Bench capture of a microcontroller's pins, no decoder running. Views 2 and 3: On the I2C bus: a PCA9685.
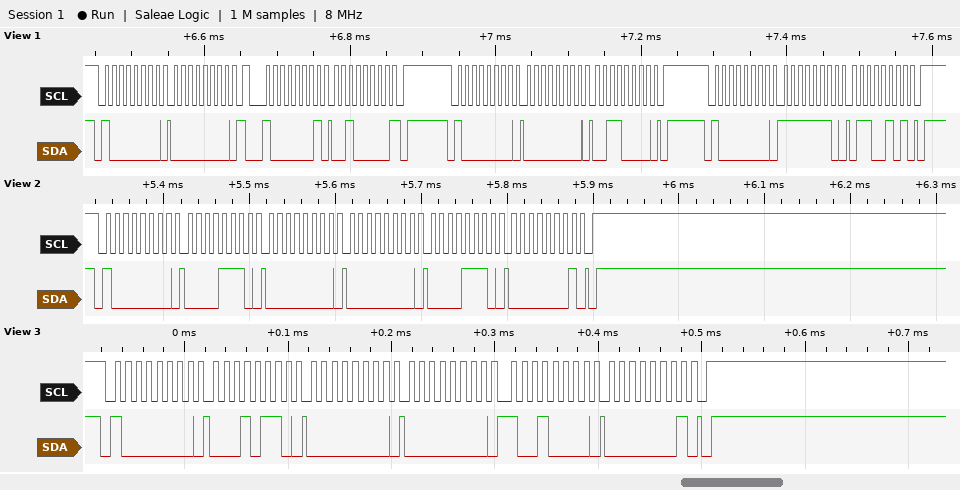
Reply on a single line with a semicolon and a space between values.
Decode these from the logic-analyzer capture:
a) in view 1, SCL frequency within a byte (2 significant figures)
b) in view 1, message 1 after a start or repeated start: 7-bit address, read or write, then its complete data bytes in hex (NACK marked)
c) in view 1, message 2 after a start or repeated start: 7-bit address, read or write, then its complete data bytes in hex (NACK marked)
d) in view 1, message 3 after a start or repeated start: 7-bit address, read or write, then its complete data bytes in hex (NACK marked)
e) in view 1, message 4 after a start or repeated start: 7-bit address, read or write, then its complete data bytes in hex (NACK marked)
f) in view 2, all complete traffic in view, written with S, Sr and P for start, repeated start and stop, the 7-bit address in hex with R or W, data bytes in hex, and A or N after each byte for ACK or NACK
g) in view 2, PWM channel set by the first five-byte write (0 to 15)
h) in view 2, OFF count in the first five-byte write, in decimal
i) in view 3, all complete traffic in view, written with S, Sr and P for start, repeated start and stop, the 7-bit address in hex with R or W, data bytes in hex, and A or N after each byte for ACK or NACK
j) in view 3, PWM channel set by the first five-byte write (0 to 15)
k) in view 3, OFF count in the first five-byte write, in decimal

100 kHz; 0x40 write: 00; 0x40 read: 20 NACK; 0x40 write: 00 30; 0x40 write: FE 65; S 40W A 0E A 00 A 00 A 0E A 01 A P; 2; 270; S 40W A 16 A 00 A 00 A 90 A 01 A P; 4; 400
